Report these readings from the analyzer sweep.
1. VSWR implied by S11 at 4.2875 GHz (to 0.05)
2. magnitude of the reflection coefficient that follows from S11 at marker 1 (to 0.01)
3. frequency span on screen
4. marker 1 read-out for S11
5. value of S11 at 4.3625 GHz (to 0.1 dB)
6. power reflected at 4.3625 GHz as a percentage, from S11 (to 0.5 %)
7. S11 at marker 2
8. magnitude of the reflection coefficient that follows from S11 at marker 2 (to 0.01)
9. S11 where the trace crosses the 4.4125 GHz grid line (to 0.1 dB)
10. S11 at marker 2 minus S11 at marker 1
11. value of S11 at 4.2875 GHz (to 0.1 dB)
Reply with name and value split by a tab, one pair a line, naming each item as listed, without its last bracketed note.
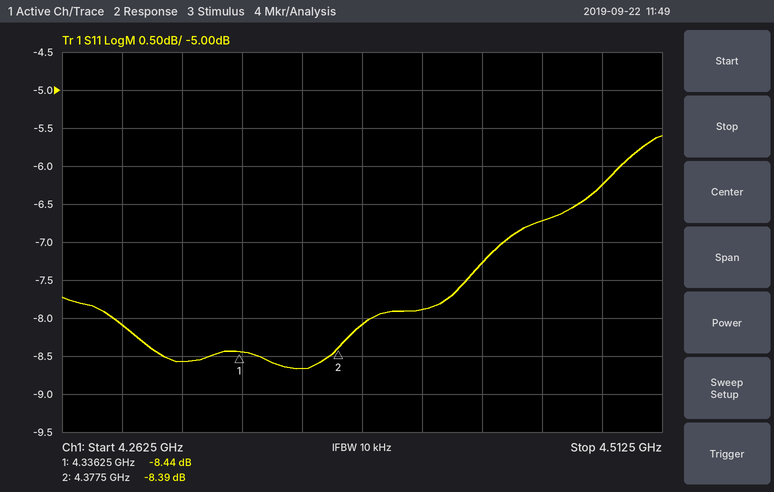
VSWR implied by S11 at 4.2875 GHz	2.30
magnitude of the reflection coefficient that follows from S11 at marker 1	0.38
frequency span on screen	250 MHz
marker 1 read-out for S11	-8.44 dB
value of S11 at 4.3625 GHz	-8.7 dB
power reflected at 4.3625 GHz as a percentage, from S11	13.5 %
S11 at marker 2	-8.39 dB
magnitude of the reflection coefficient that follows from S11 at marker 2	0.38
S11 where the trace crosses the 4.4125 GHz grid line	-7.9 dB
S11 at marker 2 minus S11 at marker 1	0.05 dB
value of S11 at 4.2875 GHz	-8.1 dB
